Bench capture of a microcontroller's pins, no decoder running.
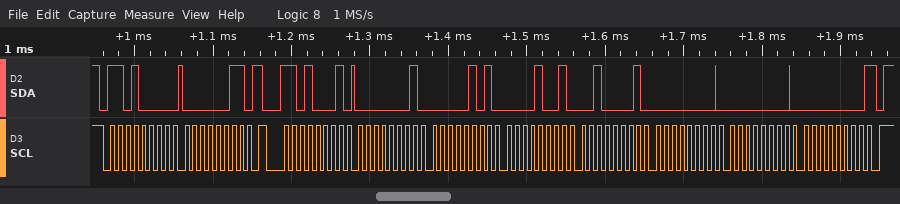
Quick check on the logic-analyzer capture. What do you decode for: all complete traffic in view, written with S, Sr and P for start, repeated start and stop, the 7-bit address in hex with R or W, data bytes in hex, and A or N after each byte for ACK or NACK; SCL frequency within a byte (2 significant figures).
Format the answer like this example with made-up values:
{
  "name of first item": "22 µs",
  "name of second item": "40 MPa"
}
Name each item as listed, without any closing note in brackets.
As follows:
{
  "all complete traffic in view, written with S, Sr and P for start, repeated start and stop, the 7-bit address in hex with R or W, data bytes in hex, and A or N after each byte for ACK or NACK": "S 68W A 03 A Sr 68R A 01 A 05 A 09 A 21 A 00 A 00 A 00 N P",
  "SCL frequency within a byte": "100 kHz"
}
